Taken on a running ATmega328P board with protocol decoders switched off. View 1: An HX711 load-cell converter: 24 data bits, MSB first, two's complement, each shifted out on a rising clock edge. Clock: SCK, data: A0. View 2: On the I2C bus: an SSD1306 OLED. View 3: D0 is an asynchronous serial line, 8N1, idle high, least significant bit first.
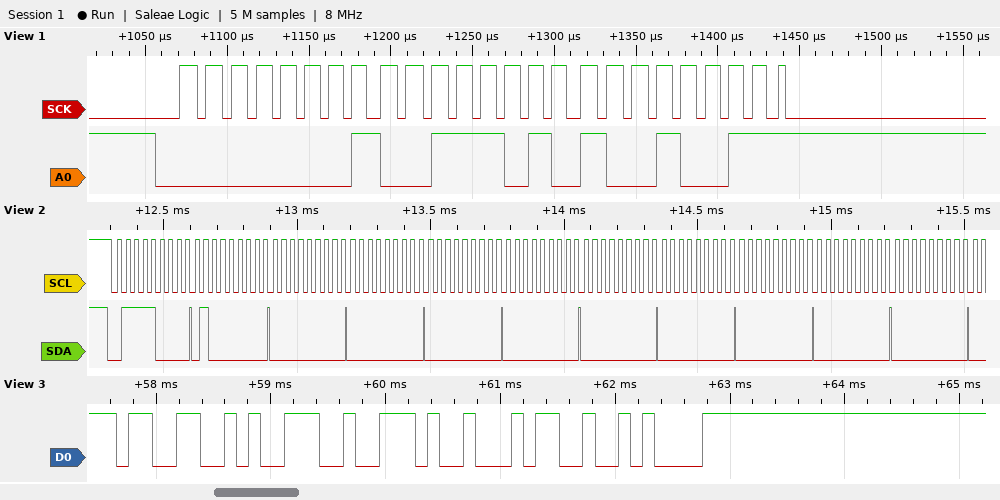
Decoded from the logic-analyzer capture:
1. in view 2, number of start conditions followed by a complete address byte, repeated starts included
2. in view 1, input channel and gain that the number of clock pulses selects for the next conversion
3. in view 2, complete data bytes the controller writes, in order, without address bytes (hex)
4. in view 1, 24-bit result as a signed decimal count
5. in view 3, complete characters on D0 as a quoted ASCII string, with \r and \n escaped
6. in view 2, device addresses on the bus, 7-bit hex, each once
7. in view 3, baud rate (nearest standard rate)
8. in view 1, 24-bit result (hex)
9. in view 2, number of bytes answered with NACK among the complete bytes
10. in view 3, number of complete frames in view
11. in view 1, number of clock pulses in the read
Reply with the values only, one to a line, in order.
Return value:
1
channel A, gain 128
40 00 00 00 00 00 00 00 00 00
80531
"39.4\n"
0x3C
9600 baud
0x013A93
0
5
25
